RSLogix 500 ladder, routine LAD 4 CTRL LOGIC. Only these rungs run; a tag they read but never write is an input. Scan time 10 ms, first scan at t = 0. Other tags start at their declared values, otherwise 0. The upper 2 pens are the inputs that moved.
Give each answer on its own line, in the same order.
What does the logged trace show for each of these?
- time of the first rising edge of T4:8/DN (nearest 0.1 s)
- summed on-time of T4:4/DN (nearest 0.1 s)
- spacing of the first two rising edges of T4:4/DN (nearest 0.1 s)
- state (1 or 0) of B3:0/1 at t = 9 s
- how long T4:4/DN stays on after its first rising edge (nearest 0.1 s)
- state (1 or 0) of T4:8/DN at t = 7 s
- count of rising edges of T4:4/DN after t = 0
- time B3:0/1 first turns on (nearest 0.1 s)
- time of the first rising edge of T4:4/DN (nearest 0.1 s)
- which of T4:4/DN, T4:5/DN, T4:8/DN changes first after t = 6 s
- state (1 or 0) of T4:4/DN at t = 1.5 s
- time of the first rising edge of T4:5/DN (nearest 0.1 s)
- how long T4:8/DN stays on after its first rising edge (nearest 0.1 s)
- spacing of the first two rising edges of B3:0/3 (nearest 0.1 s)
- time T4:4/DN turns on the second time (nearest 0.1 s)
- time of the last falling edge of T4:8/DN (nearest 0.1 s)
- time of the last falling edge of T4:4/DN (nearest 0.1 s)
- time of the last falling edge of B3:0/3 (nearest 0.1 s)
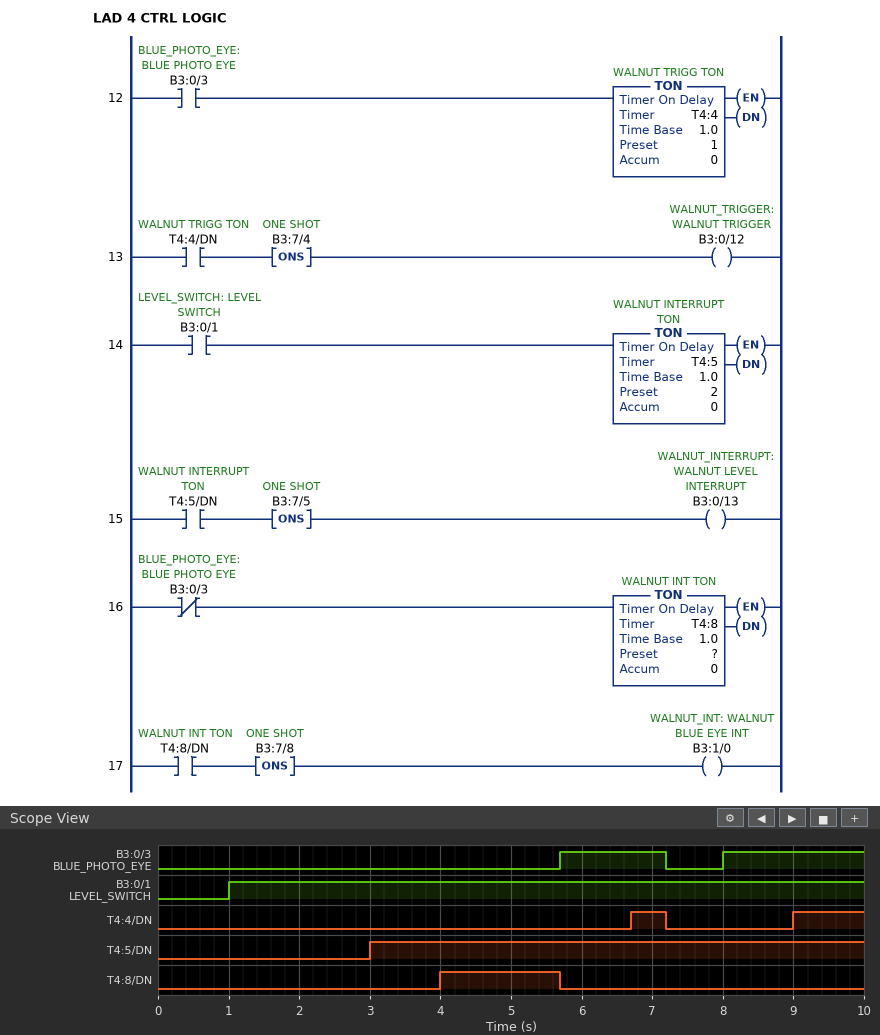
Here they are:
4.0 s
1.5 s
2.3 s
1
0.5 s
0
2
1.0 s
6.7 s
T4:4/DN
0
3.0 s
1.7 s
2.3 s
9.0 s
5.7 s
7.2 s
7.2 s
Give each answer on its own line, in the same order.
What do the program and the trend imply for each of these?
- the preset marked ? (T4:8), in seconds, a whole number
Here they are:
4 s
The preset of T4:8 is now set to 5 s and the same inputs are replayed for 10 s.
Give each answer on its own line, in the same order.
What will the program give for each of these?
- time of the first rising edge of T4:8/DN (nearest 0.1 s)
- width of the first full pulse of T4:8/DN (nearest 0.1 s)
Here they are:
5.0 s
0.7 s
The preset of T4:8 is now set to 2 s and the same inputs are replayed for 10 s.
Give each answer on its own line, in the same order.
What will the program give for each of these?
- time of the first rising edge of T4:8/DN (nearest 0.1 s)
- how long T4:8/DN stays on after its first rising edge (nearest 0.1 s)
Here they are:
2.0 s
3.7 s
